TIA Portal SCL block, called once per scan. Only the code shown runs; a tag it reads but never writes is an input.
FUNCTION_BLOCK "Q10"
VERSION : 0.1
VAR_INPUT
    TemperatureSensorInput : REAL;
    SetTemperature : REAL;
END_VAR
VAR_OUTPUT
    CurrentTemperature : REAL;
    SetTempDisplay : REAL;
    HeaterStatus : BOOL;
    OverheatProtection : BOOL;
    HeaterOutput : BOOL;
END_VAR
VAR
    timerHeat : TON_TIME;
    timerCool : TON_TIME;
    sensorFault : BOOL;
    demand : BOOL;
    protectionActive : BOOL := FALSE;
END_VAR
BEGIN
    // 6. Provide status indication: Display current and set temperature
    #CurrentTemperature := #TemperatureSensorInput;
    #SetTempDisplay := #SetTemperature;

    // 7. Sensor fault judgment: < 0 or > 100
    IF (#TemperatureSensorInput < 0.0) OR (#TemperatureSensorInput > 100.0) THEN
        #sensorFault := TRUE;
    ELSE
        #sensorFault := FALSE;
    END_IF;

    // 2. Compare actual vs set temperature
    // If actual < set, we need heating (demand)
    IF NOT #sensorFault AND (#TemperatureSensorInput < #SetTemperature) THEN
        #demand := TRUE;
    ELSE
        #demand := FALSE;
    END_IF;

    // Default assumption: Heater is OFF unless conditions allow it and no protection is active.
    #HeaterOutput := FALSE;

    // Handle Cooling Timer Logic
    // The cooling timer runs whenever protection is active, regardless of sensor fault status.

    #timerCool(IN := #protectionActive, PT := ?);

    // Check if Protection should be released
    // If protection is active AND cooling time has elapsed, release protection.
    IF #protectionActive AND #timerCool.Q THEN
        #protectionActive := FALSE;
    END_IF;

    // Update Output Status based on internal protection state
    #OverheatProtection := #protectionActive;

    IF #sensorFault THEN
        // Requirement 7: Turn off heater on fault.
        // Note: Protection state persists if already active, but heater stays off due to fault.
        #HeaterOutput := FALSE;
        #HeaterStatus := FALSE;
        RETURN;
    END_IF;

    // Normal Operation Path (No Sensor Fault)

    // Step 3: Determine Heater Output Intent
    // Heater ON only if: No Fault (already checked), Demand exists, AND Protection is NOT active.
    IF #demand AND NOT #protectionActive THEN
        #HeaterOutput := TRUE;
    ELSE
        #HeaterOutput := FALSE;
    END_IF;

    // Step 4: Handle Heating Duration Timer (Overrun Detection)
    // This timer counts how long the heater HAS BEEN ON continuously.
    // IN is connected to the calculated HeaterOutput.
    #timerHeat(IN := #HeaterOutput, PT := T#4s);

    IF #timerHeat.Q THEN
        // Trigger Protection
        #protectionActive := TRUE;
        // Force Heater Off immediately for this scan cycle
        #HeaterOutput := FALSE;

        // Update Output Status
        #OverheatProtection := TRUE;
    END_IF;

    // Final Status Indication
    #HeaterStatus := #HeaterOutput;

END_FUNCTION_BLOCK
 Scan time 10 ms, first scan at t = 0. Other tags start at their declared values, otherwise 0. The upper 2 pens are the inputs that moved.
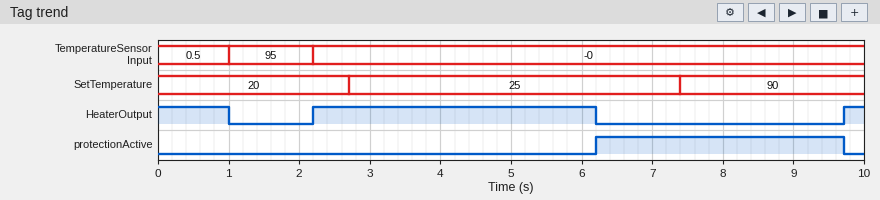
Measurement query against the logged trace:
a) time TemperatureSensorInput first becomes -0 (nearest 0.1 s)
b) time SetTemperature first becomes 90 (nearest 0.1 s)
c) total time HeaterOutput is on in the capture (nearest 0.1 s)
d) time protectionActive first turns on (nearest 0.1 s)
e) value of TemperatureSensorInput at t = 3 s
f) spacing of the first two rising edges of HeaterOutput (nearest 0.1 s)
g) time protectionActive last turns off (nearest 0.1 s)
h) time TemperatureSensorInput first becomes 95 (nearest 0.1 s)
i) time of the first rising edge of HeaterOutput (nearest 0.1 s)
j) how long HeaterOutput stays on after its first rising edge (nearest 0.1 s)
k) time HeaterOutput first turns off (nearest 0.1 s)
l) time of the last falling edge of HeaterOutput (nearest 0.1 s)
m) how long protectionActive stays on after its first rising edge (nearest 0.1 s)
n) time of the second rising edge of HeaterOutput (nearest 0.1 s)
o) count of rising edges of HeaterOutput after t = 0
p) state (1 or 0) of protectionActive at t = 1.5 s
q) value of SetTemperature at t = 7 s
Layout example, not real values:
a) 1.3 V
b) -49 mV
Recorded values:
a) 2.2 s
b) 7.4 s
c) 5.3 s
d) 6.2 s
e) -0
f) 7.5 s
g) 9.7 s
h) 1.0 s
i) 2.2 s
j) 4.0 s
k) 1.0 s
l) 6.2 s
m) 3.5 s
n) 9.7 s
o) 2
p) 0
q) 25
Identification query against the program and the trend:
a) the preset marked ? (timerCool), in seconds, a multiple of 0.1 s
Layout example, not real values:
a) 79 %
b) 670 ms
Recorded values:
a) 3.5 s
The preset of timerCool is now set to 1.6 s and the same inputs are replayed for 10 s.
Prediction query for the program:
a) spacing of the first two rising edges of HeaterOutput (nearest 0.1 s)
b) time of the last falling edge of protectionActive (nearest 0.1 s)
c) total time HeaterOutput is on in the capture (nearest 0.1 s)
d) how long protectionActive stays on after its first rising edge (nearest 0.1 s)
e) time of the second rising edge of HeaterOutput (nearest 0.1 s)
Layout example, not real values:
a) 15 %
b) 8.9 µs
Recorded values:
a) 5.6 s
b) 7.8 s
c) 7.2 s
d) 1.6 s
e) 7.8 s
